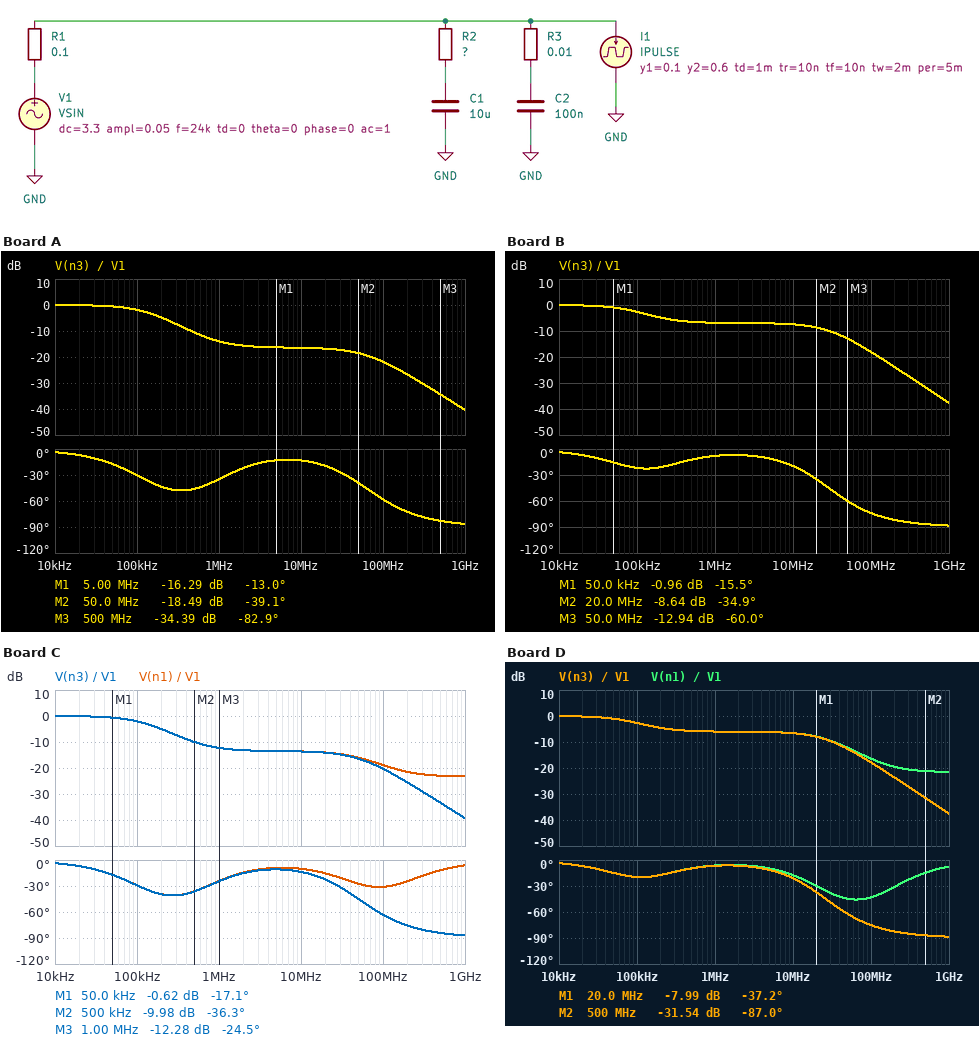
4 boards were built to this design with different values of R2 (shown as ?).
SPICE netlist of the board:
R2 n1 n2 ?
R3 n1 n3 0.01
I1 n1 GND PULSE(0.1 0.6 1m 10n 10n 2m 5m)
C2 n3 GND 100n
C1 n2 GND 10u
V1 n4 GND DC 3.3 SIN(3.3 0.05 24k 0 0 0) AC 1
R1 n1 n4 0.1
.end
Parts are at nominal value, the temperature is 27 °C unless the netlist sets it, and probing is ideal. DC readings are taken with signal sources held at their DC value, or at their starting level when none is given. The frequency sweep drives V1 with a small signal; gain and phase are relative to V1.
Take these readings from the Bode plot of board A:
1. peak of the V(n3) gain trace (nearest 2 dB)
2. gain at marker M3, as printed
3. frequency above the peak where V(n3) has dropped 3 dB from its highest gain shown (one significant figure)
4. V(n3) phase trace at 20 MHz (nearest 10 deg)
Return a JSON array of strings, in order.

["0 dB", "-34.39 dB", "100 kHz", "-20 deg"]
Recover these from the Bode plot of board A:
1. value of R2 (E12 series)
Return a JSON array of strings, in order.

["0.018 Ω"]
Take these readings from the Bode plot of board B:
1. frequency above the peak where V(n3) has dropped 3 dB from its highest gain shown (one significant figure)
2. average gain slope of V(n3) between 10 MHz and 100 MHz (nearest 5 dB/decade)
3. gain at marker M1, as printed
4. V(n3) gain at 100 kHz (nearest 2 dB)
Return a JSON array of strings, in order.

["100 kHz", "-10 dB/decade", "-0.96 dB", "-2 dB"]
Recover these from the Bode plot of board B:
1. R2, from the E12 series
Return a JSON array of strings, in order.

["0.082 Ω"]
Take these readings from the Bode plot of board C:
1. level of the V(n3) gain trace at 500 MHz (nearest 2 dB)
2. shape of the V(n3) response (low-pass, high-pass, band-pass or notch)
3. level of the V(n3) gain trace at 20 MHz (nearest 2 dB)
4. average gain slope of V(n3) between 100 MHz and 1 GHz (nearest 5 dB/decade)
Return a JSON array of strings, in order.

["-34 dB", "low-pass", "-14 dB", "-20 dB/decade"]
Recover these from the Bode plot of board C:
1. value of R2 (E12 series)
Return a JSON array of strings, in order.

["0.027 Ω"]
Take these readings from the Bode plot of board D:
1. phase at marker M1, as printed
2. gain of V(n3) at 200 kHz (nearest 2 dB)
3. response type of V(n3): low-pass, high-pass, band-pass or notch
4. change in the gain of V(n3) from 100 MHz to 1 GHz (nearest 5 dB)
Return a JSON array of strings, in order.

["-37.2 deg", "-4 dB", "low-pass", "-20 dB"]
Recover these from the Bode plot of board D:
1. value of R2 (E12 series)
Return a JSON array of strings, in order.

["0.1 Ω"]
